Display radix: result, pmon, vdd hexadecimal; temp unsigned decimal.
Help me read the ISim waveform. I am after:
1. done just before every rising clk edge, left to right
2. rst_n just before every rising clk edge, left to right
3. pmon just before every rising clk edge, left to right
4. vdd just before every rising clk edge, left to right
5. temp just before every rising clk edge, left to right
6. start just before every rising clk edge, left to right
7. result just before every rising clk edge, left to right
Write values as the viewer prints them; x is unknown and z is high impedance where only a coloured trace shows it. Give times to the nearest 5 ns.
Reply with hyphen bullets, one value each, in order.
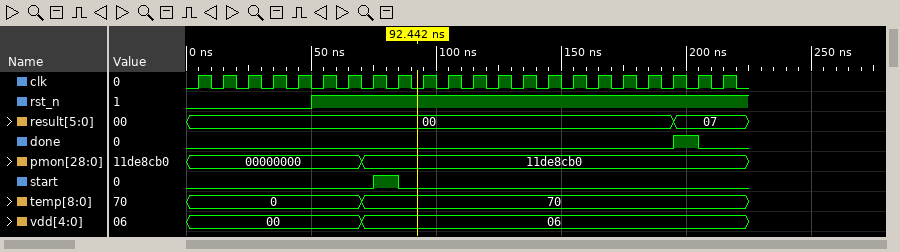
- 0 0 0 0 0 0 0 0 0 0 0 0 0 0 0 0 0 0 0 0 1 0
- 0 0 0 0 0 1 1 1 1 1 1 1 1 1 1 1 1 1 1 1 1 1
- 00000000, 00000000, 00000000, 00000000, 00000000, 00000000, 00000000, 11de8cb0, 11de8cb0, 11de8cb0, 11de8cb0, 11de8cb0, 11de8cb0, 11de8cb0, 11de8cb0, 11de8cb0, 11de8cb0, 11de8cb0, 11de8cb0, 11de8cb0, 11de8cb0, 11de8cb0
- 00, 00, 00, 00, 00, 00, 00, 06, 06, 06, 06, 06, 06, 06, 06, 06, 06, 06, 06, 06, 06, 06
- 0, 0, 0, 0, 0, 0, 0, 70, 70, 70, 70, 70, 70, 70, 70, 70, 70, 70, 70, 70, 70, 70
- 0 0 0 0 0 0 0 0 1 0 0 0 0 0 0 0 0 0 0 0 0 0
- 00, 00, 00, 00, 00, 00, 00, 00, 00, 00, 00, 00, 00, 00, 00, 00, 00, 00, 00, 00, 07, 07
